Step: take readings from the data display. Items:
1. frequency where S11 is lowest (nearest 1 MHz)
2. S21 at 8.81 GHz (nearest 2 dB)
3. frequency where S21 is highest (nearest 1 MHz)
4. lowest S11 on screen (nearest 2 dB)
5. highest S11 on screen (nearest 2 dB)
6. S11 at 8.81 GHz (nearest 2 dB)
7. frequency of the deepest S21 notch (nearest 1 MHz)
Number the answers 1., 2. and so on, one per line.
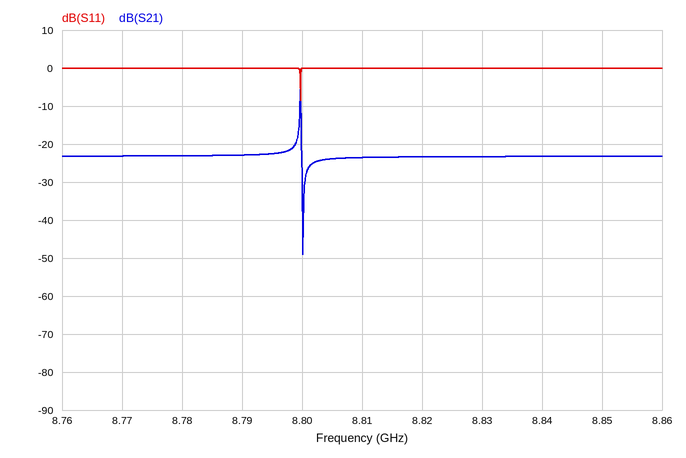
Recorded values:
1. 8.800 GHz
2. -24 dB
3. 8.800 GHz
4. -8 dB
5. 0 dB
6. 0 dB
7. 8.800 GHz
